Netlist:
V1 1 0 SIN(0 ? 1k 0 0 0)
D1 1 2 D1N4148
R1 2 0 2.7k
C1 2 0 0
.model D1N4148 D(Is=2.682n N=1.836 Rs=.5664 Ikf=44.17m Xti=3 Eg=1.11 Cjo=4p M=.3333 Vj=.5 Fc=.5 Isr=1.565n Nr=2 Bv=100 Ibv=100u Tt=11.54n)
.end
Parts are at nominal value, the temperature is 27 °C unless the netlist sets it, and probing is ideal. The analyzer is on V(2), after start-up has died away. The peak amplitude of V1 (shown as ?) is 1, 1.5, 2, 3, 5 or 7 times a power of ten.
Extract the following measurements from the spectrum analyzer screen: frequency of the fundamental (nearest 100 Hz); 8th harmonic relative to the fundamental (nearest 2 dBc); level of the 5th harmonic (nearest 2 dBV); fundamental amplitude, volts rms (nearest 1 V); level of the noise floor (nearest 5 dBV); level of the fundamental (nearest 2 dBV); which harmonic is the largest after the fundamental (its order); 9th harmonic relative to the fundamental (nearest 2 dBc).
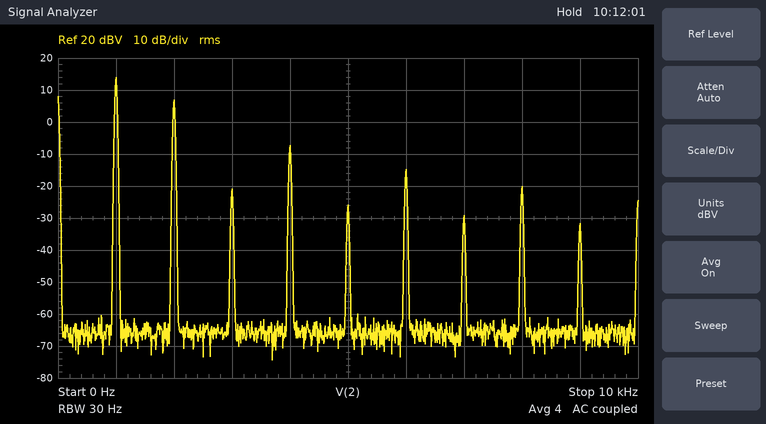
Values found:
1.0 kHz
-34 dBc
-26 dBV
5 V
-65 dBV
14 dBV
2
-46 dBc
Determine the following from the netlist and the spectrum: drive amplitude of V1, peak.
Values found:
15 V
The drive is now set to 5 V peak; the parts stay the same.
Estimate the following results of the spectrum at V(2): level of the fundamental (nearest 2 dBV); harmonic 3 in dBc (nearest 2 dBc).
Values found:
4 dBV
-26 dBc
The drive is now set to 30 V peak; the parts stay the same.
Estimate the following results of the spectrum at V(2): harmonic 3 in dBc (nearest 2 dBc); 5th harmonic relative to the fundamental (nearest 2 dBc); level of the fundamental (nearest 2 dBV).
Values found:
-40 dBc
-46 dBc
20 dBV
